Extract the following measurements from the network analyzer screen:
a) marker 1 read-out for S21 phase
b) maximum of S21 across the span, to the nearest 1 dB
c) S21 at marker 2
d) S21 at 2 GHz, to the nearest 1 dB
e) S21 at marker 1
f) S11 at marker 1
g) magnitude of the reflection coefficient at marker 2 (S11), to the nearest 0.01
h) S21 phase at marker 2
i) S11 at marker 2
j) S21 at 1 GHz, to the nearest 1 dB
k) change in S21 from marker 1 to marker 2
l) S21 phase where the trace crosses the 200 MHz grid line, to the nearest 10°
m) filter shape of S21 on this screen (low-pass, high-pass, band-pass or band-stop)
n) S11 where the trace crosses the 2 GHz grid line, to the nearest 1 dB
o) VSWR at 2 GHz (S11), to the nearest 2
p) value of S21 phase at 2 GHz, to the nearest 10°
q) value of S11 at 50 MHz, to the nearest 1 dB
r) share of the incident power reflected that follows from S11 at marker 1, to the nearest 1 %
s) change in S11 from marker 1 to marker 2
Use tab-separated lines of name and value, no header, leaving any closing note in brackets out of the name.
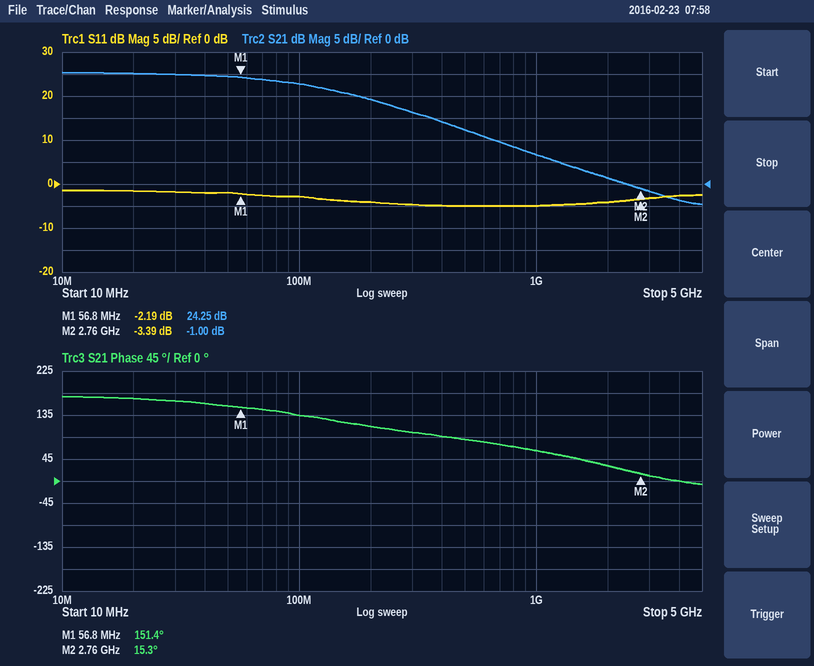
marker 1 read-out for S21 phase	151.4°
maximum of S21 across the span, to the nearest 1 dB	25 dB
S21 at marker 2	-1.00 dB
S21 at 2 GHz, to the nearest 1 dB	1 dB
S21 at marker 1	24.25 dB
S11 at marker 1	-2.19 dB
magnitude of the reflection coefficient at marker 2 (S11), to the nearest 0.01	0.68
S21 phase at marker 2	15.3°
S11 at marker 2	-3.39 dB
S21 at 1 GHz, to the nearest 1 dB	7 dB
change in S21 from marker 1 to marker 2	-25.25 dB
S21 phase where the trace crosses the 200 MHz grid line, to the nearest 10°	110°
filter shape of S21 on this screen	low-pass
S11 where the trace crosses the 2 GHz grid line, to the nearest 1 dB	-4 dB
VSWR at 2 GHz (S11), to the nearest 2	4
value of S21 phase at 2 GHz, to the nearest 10°	30°
value of S11 at 50 MHz, to the nearest 1 dB	-2 dB
share of the incident power reflected that follows from S11 at marker 1, to the nearest 1 %	60 %
change in S11 from marker 1 to marker 2	-1.20 dB
